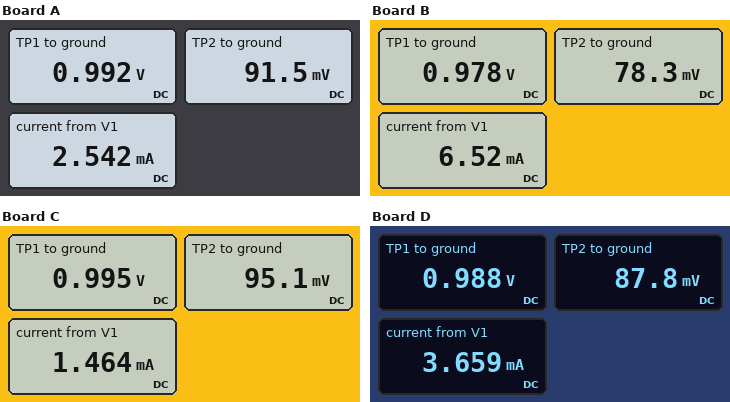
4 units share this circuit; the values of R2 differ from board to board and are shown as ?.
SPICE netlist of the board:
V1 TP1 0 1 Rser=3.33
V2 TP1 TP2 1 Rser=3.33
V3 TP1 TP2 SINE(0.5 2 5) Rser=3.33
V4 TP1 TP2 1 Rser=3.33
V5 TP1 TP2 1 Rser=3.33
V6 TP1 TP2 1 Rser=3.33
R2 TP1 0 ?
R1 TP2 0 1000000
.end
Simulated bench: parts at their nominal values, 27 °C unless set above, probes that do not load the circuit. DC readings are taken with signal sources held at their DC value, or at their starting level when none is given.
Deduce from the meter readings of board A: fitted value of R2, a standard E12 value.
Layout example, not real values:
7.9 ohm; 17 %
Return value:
390 Ω
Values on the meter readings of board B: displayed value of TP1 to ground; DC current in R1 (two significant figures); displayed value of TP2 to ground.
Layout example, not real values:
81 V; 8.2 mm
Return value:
0.978 V; 78 nA; 78.3 mV
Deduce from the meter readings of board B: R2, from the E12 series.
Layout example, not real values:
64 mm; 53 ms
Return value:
150 Ω
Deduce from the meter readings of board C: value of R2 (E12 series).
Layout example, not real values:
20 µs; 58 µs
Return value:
680 Ω
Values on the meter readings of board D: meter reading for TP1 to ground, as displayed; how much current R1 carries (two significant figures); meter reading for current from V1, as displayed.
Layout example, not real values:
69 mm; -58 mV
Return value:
0.988 V; 88 nA; 3.659 mA
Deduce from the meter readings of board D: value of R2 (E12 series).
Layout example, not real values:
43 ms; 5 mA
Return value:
270 Ω
